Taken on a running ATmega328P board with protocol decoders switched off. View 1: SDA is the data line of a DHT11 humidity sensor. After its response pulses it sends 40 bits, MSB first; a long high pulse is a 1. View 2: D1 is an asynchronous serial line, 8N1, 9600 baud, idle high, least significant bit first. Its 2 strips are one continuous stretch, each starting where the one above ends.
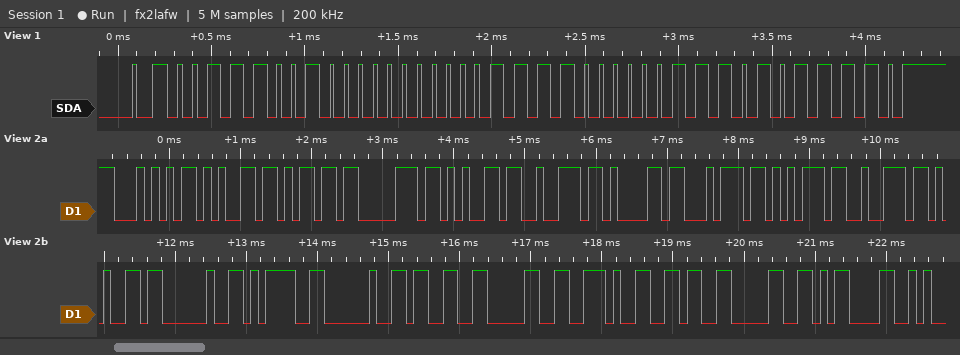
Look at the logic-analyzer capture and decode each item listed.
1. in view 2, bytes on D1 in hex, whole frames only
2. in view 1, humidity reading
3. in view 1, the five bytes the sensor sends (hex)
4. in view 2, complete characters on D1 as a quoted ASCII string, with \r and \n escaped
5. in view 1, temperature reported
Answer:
54 65 6D 70 65 72 61 74 75 72 65 20 3D 20 33 30 2E 36 30 0D
57 %
39 00 1E 07 5E
"Temperature = 30.60\r"
30.7 °C
